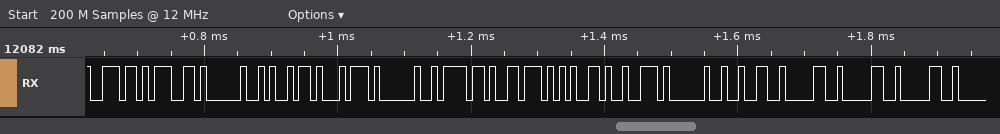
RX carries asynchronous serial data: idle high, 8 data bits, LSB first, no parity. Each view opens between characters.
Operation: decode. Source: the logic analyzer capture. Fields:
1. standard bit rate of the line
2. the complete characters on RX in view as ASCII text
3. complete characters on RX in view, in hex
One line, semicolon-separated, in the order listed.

115200 baud; "ng it over 2000"; 6E, 67, 20, 69, 74, 20, 6F, 76, 65, 72, 20, 32, 30, 30, 30
